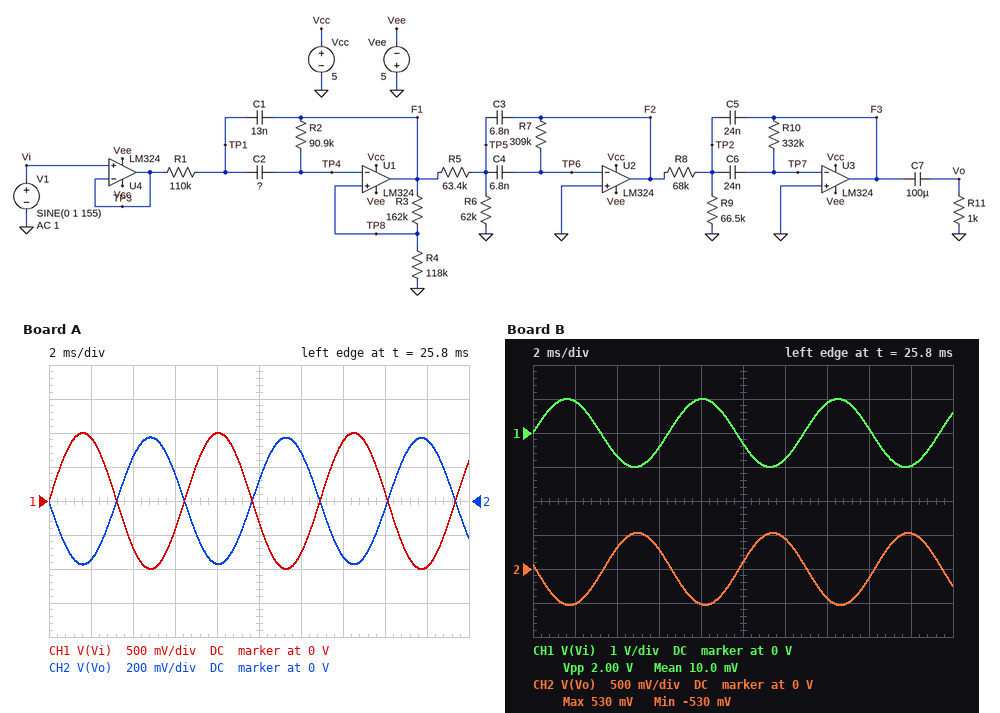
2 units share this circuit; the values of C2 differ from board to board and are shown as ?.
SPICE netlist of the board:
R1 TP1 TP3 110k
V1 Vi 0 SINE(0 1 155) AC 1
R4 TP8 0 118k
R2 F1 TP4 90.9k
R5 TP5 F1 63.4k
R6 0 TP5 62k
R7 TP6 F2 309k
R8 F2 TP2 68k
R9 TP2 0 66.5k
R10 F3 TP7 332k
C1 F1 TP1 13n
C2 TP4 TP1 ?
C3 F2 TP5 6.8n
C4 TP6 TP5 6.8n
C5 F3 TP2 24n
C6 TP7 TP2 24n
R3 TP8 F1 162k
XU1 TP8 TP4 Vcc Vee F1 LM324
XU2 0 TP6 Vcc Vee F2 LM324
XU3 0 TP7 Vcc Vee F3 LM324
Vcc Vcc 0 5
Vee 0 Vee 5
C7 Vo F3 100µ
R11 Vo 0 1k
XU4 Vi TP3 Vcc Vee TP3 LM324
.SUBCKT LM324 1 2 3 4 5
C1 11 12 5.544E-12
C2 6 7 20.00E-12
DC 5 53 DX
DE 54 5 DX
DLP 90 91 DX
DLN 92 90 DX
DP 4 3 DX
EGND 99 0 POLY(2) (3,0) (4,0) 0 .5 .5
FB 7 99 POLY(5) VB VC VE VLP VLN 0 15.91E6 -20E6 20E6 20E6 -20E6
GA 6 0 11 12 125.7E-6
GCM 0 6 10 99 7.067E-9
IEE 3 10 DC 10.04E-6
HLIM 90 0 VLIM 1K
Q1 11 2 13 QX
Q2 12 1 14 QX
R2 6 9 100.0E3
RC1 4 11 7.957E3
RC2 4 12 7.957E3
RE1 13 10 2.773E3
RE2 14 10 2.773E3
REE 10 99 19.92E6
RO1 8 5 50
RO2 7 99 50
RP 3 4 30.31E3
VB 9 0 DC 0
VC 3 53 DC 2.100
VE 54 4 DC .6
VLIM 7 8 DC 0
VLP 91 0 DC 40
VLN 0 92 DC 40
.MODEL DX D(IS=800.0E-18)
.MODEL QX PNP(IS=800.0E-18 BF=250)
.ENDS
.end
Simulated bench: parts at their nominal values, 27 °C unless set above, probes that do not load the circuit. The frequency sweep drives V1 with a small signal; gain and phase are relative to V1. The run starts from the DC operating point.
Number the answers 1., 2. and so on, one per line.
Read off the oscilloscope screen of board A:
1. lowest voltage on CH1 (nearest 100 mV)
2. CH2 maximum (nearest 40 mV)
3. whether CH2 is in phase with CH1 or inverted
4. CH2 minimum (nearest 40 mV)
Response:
1. -1.0 V
2. 360 mV
3. inverted
4. -360 mV
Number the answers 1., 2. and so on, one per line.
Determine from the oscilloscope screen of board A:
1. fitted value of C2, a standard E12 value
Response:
1. 3.9 nF
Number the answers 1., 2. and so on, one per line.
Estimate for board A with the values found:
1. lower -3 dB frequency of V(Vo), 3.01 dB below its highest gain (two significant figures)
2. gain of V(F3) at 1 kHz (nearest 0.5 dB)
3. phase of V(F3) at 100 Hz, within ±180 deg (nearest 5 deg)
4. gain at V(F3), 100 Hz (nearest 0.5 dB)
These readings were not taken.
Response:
1. 100 Hz
2. -43.5 dB
3. -125 deg
4. -10.5 dB
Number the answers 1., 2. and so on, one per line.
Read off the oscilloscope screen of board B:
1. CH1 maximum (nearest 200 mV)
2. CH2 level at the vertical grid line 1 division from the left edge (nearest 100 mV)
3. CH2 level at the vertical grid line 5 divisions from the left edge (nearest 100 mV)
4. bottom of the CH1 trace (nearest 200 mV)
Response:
1. 1.0 V
2. -500 mV
3. 100 mV
4. -1.0 V
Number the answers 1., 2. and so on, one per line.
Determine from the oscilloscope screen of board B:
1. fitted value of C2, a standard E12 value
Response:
1. 5.6 nF
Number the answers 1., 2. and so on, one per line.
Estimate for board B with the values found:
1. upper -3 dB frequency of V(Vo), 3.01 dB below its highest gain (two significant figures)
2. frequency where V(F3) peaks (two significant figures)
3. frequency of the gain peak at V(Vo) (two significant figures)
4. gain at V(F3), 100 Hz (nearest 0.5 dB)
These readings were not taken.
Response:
1. 270 Hz
2. 200 Hz
3. 200 Hz
4. -7.0 dB
